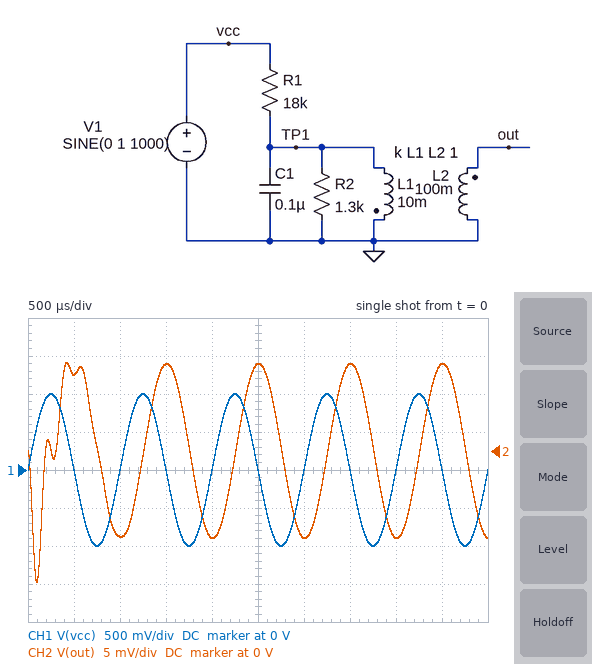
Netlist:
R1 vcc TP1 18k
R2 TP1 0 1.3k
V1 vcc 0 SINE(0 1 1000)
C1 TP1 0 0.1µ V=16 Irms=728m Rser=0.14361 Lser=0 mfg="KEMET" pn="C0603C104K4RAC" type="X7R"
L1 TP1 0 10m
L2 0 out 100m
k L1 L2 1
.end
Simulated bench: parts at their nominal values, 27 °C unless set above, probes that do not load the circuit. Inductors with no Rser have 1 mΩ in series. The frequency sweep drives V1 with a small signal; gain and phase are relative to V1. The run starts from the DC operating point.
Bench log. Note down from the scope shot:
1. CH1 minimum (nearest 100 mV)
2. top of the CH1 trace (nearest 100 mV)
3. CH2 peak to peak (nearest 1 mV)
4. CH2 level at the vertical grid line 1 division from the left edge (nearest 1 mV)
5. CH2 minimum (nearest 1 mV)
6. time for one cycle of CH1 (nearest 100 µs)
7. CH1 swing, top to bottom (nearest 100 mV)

-1.0 V
1.0 V
29 mV
10 mV
-17 mV
1.0 ms
2.0 V
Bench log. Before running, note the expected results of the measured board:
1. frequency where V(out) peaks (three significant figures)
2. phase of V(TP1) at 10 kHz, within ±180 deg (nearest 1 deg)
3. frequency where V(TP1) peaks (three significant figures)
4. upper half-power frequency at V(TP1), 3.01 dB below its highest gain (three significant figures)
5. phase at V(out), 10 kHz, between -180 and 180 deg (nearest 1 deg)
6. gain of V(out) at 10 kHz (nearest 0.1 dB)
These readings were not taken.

5.03 kHz
-80 deg
5.03 kHz
5.73 kHz
100 deg
-28.7 dB
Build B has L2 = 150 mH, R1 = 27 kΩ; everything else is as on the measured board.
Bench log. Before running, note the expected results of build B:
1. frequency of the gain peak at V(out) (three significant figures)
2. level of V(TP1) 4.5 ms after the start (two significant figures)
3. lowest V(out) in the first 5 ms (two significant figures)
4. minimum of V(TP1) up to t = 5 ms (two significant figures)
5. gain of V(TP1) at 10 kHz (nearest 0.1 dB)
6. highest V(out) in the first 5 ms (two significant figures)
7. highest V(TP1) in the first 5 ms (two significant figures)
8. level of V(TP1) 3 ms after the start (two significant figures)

5.03 kHz
-2.4 mV
-14 mV
-2.5 mV
-42.2 dB
9.5 mV
3.7 mV
2.4 mV
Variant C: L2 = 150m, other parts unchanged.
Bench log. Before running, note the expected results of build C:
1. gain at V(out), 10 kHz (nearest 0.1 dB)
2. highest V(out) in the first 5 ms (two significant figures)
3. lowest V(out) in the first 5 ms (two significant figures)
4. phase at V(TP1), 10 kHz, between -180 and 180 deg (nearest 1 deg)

-26.9 dB
14 mV
-21 mV
-80 deg
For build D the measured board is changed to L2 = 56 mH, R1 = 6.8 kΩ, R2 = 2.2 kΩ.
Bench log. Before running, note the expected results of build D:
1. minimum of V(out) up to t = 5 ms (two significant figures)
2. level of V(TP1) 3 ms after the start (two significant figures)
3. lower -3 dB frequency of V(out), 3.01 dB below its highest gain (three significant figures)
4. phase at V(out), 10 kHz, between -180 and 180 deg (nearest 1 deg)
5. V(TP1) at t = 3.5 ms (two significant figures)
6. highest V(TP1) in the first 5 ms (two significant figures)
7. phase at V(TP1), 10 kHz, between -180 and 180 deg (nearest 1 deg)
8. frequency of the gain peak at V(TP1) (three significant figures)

-36 mV
9.6 mV
4.58 kHz
97 deg
-9.6 mV
15 mV
-83 deg
5.03 kHz
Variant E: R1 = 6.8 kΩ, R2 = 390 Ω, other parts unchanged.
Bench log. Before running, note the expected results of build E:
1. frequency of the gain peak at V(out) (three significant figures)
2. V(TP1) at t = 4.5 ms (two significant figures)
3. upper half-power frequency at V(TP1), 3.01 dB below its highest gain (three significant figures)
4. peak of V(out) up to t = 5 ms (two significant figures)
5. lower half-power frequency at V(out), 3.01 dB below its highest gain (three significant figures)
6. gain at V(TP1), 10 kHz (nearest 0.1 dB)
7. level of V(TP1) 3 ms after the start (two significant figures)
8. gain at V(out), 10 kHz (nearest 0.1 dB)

5.03 kHz
-9.3 mV
7.63 kHz
30 mV
3.32 kHz
-31.3 dB
9.3 mV
-21.3 dB
